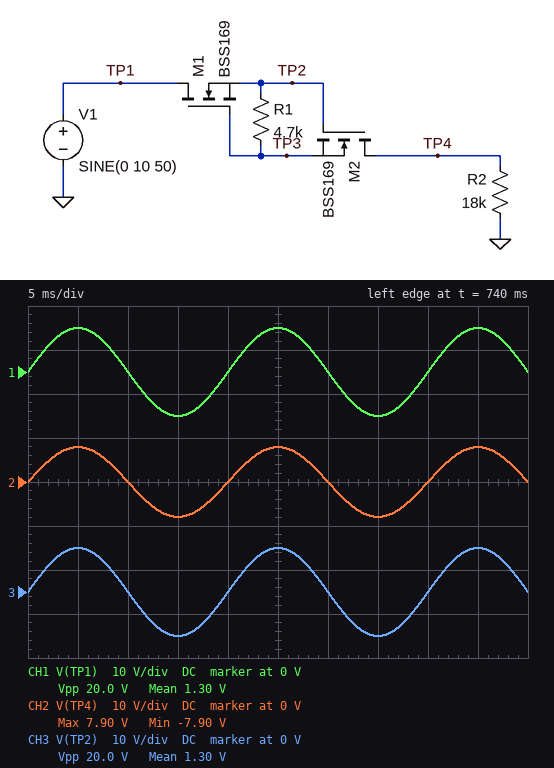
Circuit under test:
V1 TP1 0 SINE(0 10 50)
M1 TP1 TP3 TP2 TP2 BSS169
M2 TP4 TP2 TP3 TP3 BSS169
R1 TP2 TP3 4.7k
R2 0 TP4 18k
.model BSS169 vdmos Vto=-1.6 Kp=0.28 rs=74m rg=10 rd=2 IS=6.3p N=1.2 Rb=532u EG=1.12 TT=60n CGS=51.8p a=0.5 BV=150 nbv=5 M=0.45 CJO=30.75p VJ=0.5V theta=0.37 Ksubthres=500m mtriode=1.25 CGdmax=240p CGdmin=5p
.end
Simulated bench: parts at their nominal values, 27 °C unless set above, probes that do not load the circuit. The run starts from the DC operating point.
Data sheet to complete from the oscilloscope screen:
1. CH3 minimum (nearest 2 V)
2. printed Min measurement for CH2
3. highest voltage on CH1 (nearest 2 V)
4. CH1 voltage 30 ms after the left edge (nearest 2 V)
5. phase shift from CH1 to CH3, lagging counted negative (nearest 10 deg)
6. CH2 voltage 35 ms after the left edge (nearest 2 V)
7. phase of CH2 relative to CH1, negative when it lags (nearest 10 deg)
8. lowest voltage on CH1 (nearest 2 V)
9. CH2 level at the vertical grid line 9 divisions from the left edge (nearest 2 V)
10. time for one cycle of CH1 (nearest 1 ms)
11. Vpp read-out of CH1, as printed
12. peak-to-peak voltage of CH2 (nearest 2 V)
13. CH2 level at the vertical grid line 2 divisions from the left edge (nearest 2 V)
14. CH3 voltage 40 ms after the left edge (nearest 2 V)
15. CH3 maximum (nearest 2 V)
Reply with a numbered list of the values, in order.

1. -10 V
2. -7.90 V
3. 10 V
4. 0 V
5. 0 deg
6. -8 V
7. 0 deg
8. -10 V
9. 8 V
10. 20 ms
11. 20.0 V
12. 16 V
13. 0 V
14. 0 V
15. 10 V
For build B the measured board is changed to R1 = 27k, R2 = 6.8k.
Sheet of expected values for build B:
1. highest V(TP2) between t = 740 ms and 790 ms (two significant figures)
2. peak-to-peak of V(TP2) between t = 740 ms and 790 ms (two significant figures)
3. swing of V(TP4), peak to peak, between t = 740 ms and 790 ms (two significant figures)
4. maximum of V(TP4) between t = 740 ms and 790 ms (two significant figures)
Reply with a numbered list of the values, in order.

1. 3.8 V
2. 14 V
3. 1.5 V
4. 770 mV
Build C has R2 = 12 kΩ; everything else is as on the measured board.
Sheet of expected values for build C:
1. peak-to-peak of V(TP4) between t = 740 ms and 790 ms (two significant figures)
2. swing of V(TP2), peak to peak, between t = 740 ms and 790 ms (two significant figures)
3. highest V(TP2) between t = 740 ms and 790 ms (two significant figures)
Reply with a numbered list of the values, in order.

1. 13 V
2. 19 V
3. 9.3 V
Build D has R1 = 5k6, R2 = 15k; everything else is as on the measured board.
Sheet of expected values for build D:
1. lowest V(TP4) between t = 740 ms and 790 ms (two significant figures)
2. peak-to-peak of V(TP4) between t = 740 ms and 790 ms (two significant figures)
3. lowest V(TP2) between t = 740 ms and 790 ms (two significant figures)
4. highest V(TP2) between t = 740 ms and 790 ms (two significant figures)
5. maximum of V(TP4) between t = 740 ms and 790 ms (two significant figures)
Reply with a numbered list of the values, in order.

1. -7.1 V
2. 14 V
3. -10 V
4. 9.7 V
5. 7.1 V
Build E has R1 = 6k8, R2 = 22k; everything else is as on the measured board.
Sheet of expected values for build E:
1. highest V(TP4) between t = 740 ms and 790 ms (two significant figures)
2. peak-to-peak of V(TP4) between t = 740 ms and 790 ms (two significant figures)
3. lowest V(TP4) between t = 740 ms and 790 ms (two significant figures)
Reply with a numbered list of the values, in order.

1. 7.6 V
2. 15 V
3. -7.6 V
